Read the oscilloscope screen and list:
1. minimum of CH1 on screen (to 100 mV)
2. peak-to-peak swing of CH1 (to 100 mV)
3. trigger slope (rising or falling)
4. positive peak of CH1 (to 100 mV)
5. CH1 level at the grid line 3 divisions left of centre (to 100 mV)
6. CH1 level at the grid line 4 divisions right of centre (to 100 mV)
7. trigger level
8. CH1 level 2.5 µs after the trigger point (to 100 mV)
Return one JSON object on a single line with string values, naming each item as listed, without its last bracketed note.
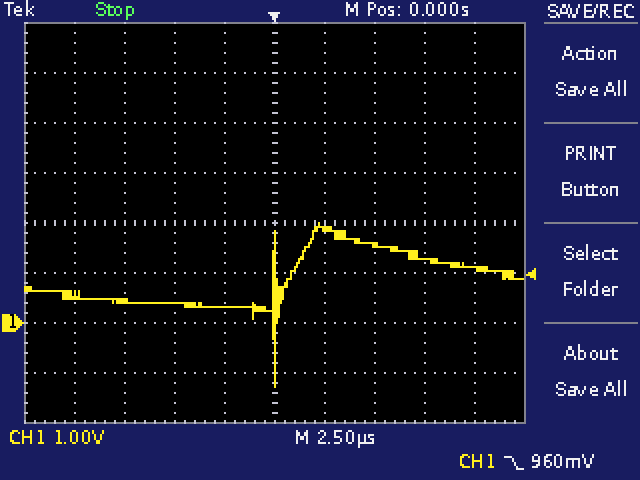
{"minimum of CH1 on screen": "-1.3 V", "peak-to-peak swing of CH1": "3.3 V", "trigger slope": "falling", "positive peak of CH1": "2.0 V", "CH1 level at the grid line 3 divisions left of centre": "400 mV", "CH1 level at the grid line 4 divisions right of centre": "1.1 V", "trigger level": "960 mV", "CH1 level 2.5 µs after the trigger point": "1.9 V"}
